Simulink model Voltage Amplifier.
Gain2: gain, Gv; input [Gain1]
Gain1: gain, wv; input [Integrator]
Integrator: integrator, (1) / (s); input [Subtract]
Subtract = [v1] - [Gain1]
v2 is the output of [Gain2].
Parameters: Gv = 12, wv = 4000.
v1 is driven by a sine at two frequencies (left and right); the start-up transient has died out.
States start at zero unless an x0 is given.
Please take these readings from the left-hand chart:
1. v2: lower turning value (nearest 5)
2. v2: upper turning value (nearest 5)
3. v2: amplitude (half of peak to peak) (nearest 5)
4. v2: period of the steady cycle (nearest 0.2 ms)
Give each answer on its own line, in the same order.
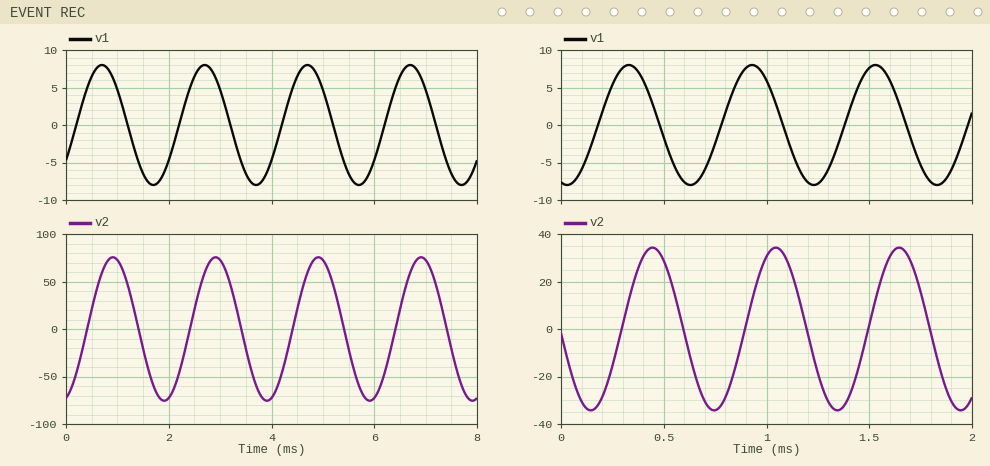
-75
75
75
2.0 ms
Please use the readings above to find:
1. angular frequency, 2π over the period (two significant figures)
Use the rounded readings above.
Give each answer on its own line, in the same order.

3.1 rad/ms
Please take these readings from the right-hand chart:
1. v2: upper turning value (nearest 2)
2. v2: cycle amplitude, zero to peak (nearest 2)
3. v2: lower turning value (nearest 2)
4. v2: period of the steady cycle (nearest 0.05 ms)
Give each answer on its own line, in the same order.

34
34
-34
0.60 ms
